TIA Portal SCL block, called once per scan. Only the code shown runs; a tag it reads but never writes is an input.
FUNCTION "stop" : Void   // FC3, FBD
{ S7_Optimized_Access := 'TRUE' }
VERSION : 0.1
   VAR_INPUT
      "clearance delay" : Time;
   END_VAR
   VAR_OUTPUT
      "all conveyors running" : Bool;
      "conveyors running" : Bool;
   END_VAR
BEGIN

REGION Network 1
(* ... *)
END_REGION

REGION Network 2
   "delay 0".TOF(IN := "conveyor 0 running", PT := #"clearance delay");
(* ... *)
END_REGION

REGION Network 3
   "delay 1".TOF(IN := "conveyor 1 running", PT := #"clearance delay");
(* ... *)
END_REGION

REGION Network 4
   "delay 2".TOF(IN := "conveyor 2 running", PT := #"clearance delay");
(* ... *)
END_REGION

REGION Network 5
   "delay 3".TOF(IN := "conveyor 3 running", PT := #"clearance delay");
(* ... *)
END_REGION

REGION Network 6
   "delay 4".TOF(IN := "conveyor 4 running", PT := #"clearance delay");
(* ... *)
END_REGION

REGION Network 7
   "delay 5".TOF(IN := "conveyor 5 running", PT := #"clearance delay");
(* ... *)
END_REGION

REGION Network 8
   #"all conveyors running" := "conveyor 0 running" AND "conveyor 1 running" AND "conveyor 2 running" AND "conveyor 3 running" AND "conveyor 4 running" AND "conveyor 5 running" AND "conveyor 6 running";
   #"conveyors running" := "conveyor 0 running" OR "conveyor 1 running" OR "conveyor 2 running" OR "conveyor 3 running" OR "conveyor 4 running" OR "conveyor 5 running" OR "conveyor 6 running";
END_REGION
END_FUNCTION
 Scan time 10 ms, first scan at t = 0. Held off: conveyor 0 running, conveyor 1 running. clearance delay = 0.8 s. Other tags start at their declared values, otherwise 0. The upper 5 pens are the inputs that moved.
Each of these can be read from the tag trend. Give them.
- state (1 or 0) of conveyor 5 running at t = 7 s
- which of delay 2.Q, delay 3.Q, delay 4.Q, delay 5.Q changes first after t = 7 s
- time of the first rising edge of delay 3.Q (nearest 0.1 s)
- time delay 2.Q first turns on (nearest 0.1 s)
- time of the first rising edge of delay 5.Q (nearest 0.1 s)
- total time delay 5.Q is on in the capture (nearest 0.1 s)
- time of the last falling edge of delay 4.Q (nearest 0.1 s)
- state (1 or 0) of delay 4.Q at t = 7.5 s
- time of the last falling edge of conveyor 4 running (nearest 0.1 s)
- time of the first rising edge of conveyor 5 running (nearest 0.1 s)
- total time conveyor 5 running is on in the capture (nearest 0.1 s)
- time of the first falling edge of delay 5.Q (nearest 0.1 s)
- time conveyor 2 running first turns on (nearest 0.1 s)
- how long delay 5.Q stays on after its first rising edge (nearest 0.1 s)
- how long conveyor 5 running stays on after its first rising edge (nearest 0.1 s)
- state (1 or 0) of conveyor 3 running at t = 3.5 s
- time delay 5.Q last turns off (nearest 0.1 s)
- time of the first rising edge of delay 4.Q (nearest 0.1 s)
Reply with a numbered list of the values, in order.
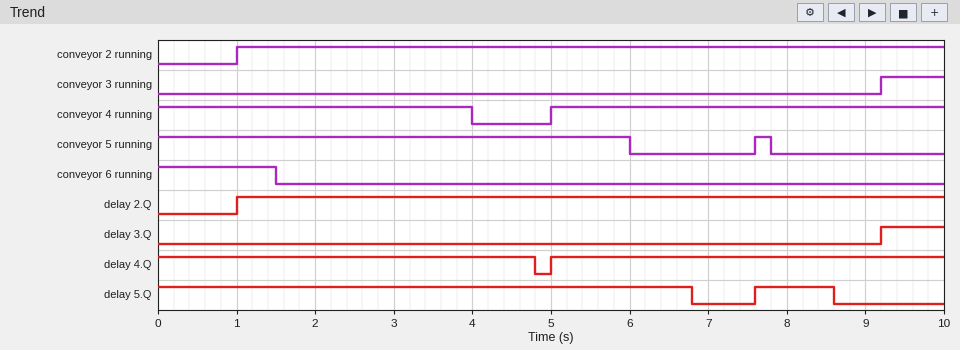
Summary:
1. 0
2. delay 5.Q
3. 9.2 s
4. 1.0 s
5. 7.6 s
6. 7.8 s
7. 4.8 s
8. 1
9. 4.0 s
10. 7.6 s
11. 6.2 s
12. 6.8 s
13. 1.0 s
14. 1.0 s
15. 0.2 s
16. 0
17. 8.6 s
18. 5.0 s
